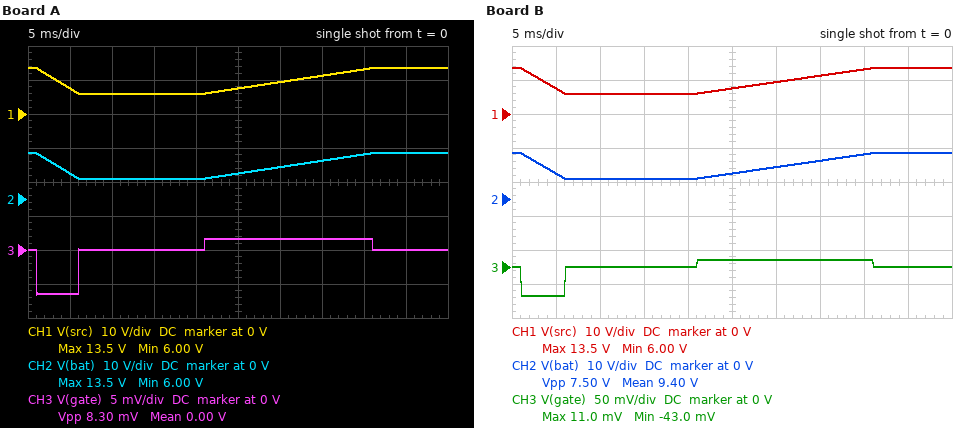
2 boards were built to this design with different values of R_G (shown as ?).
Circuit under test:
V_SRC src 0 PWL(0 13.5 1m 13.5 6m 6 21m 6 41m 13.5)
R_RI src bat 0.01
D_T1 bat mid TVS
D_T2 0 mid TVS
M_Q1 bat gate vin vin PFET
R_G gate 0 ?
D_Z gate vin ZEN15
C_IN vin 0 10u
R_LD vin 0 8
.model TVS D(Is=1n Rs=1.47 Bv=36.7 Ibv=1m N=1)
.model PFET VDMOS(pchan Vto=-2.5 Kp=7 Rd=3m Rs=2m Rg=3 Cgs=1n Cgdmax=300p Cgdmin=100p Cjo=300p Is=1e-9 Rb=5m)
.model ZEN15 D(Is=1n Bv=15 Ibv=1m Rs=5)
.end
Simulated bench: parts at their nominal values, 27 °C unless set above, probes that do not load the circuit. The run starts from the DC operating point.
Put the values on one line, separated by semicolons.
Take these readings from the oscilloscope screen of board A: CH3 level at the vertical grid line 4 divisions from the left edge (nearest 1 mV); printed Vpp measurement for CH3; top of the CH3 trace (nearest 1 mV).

0 V; 8.30 mV; 2 mV
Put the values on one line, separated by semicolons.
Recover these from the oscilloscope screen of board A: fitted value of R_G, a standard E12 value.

3.3 kΩ
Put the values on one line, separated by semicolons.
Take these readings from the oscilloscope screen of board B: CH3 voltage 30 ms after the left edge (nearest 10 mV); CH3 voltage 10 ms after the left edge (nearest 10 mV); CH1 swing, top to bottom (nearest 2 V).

10 mV; 0 V; 8 V
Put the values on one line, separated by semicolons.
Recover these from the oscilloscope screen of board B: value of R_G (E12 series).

22 kΩ
